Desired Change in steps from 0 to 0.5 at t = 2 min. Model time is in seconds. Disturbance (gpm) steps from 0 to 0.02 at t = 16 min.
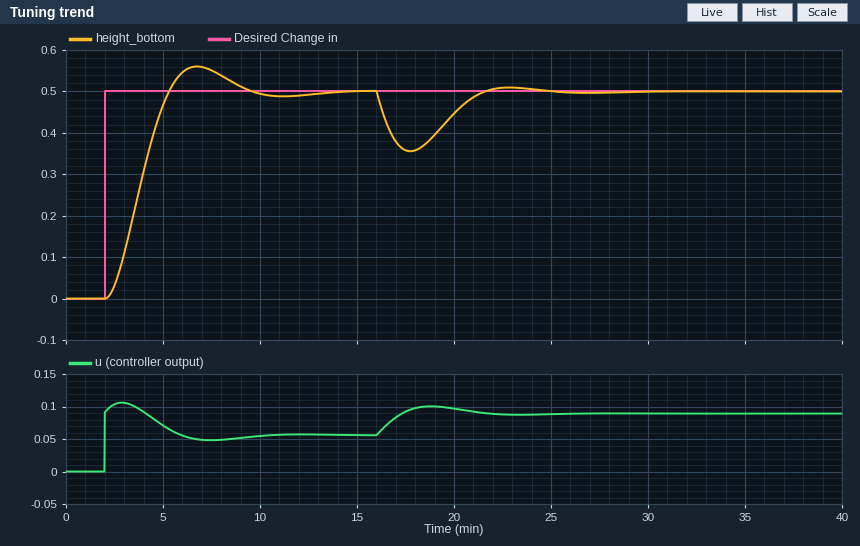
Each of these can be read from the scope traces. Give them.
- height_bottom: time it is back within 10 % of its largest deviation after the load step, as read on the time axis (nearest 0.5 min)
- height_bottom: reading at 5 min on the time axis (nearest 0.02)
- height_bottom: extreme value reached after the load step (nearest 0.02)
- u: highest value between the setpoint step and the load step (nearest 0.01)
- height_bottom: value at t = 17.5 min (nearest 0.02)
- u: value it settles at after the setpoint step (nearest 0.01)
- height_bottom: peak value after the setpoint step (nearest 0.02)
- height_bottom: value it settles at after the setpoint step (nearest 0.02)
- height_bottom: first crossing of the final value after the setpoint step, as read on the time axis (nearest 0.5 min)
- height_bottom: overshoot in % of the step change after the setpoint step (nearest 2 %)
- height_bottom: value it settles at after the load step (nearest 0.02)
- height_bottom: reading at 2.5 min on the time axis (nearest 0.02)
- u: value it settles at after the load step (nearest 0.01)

21.0 min
0.46
0.36
0.11
0.36
0.06
0.56
0.50
5.5 min
12 %
0.50
0.04
0.09
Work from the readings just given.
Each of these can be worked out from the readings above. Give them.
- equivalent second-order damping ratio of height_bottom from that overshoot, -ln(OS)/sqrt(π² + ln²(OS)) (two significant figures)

0.56
